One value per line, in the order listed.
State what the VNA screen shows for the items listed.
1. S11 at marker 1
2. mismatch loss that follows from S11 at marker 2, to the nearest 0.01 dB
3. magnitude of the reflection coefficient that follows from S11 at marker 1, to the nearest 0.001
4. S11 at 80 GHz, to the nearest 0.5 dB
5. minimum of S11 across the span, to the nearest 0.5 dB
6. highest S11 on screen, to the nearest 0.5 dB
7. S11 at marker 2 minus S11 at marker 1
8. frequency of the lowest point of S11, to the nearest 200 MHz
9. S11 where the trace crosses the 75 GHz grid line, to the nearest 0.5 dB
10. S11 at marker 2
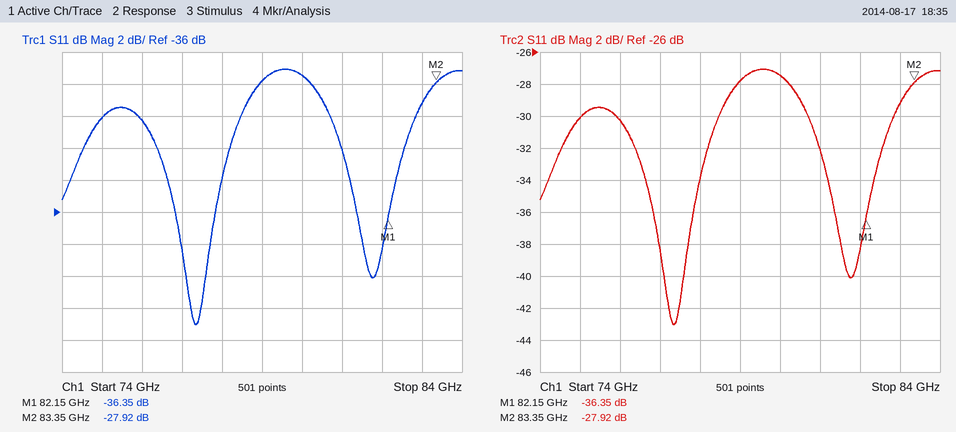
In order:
-36.35 dB
0.01 dB
0.015
-27.5 dB
-43.0 dB
-27.0 dB
8.43 dB
77.4 GHz
-30.0 dB
-27.92 dB
